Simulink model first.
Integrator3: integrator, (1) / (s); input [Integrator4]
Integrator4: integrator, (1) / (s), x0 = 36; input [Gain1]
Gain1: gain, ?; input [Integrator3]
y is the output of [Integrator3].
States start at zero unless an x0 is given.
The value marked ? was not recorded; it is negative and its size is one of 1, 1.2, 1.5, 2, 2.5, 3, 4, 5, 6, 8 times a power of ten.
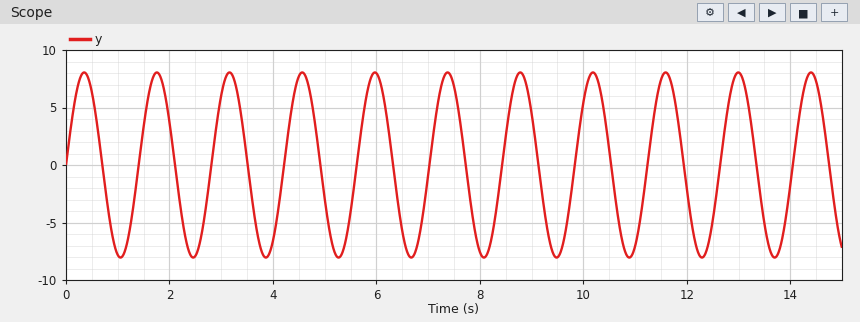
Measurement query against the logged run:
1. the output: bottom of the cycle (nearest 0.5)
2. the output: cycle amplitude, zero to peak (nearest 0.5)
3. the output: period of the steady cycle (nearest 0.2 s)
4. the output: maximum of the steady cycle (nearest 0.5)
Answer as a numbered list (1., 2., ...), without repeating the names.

1. -8.0
2. 8.0
3. 1.4 s
4. 8.0
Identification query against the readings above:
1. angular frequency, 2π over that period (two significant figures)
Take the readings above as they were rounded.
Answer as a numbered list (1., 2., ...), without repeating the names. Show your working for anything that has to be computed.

1. 2π / 1.4 = 4.5 rad/s
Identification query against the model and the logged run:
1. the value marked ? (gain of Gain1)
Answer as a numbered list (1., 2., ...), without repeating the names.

1. -20
